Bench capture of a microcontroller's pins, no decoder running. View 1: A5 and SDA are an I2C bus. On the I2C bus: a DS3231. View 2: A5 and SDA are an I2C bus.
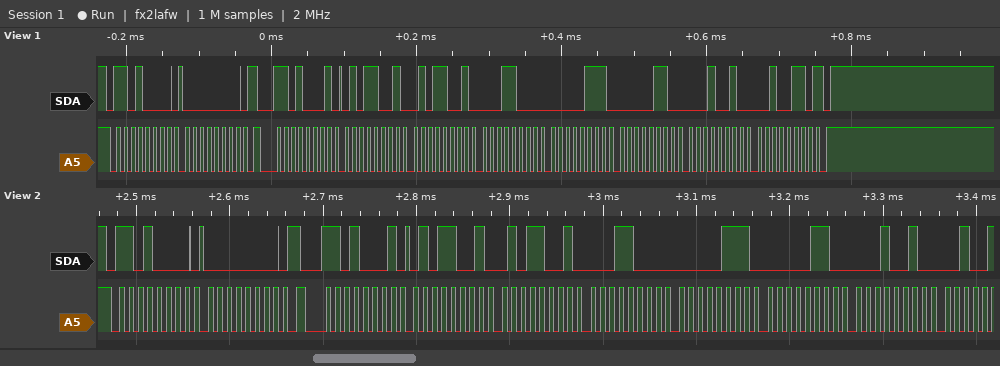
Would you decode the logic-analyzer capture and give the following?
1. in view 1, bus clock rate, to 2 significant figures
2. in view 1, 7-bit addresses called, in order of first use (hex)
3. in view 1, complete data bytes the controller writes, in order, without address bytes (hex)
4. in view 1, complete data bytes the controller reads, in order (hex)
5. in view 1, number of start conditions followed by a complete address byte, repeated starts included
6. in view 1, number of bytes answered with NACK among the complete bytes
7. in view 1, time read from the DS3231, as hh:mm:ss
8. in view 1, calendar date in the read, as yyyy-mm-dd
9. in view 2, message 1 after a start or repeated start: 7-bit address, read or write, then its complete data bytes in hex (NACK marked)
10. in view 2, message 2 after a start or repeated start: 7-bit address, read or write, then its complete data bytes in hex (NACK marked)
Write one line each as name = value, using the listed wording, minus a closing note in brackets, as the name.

in view 1, bus clock rate, to 2 significant figures = 100 kHz
in view 1, 7-bit addresses called, in order of first use = 0x68
in view 1, complete data bytes the controller writes, in order, without address bytes = 00
in view 1, complete data bytes the controller reads, in order = 59 59 18 07 06 12 26
in view 1, number of start conditions followed by a complete address byte, repeated starts included = 2
in view 1, number of bytes answered with NACK among the complete bytes = 1
in view 1, time read from the DS3231, as hh:mm:ss = 18:59:59
in view 1, calendar date in the read, as yyyy-mm-dd = 2026-12-06
in view 2, message 1 after a start or repeated start: 7-bit address, read or write, then its complete data bytes in hex = 0x68 write: 00
in view 2, message 2 after a start or repeated start: 7-bit address, read or write, then its complete data bytes in hex = 0x68 read: 59 59 18 07 06 12
